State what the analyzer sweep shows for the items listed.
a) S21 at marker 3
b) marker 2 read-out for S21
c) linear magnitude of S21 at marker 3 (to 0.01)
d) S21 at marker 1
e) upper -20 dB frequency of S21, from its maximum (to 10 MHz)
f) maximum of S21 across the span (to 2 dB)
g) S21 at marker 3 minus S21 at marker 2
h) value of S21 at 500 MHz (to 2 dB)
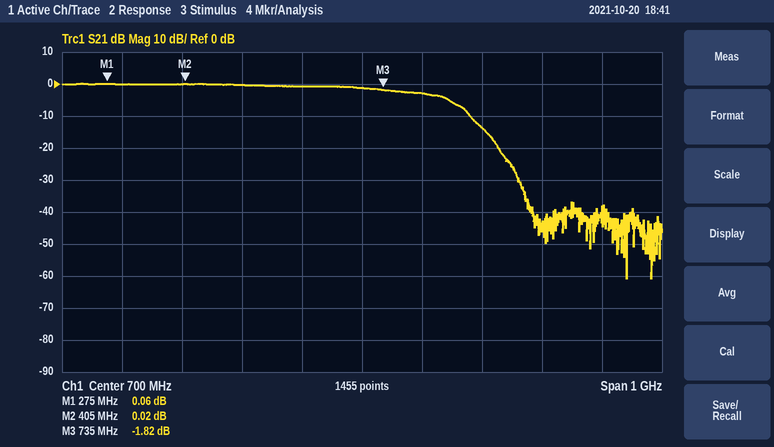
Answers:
-1.82 dB
0.02 dB
0.81
0.06 dB
930 MHz
0 dB
-1.84 dB
0 dB
